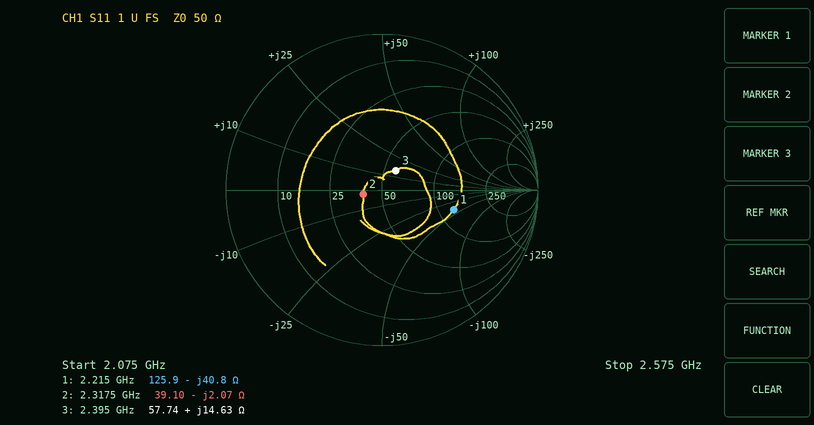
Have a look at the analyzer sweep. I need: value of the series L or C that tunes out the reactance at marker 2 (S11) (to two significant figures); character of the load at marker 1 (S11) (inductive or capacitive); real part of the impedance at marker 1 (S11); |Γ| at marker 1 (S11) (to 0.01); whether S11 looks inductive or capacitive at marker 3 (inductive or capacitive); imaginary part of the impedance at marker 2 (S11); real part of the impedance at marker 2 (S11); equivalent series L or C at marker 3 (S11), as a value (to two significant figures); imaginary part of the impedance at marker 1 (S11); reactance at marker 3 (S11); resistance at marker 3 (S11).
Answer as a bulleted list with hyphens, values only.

- 140 pH
- capacitive
- 125.9 Ω
- 0.48
- inductive
- -2.07 Ω
- 39.10 Ω
- 970 pH
- -40.8 Ω
- +14.63 Ω
- 57.74 Ω
